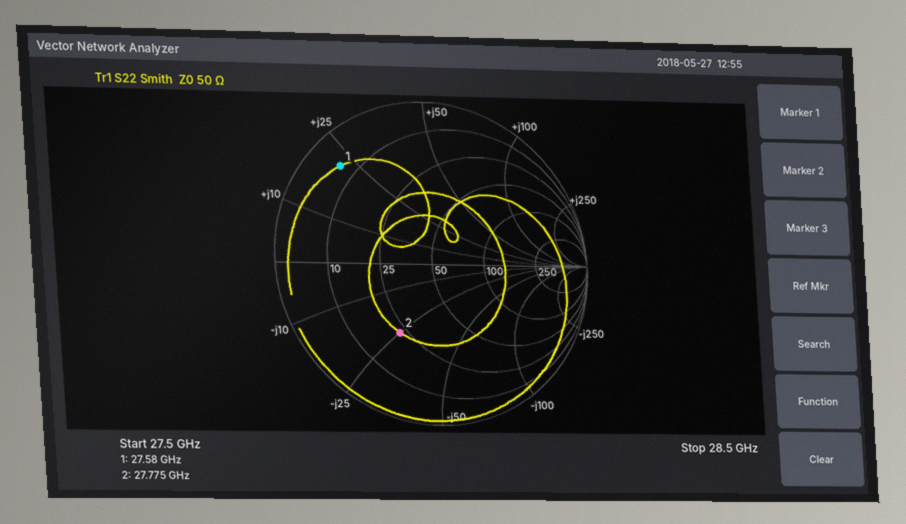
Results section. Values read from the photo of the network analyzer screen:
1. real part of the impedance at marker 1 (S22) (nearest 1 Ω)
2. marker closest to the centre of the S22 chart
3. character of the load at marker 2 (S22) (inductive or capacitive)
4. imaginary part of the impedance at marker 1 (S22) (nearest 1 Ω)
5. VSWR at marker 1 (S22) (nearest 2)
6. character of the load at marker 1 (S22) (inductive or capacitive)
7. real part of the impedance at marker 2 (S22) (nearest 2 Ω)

6 Ω
marker 2
capacitive
+22 Ω
10
inductive
22 Ω
